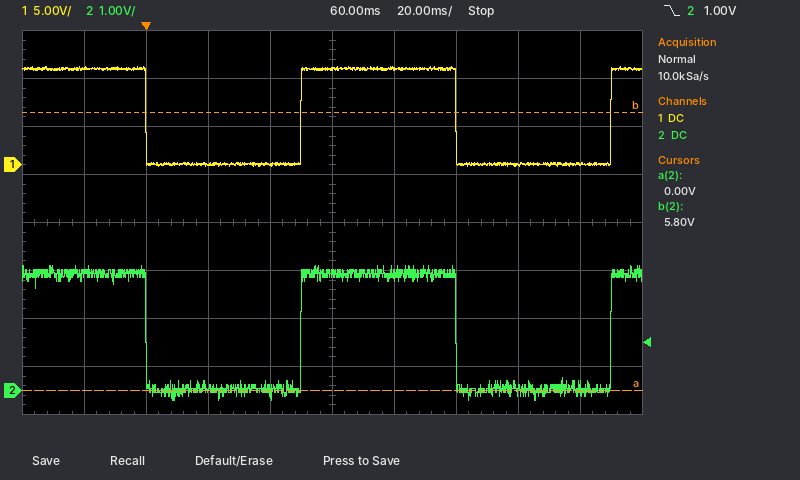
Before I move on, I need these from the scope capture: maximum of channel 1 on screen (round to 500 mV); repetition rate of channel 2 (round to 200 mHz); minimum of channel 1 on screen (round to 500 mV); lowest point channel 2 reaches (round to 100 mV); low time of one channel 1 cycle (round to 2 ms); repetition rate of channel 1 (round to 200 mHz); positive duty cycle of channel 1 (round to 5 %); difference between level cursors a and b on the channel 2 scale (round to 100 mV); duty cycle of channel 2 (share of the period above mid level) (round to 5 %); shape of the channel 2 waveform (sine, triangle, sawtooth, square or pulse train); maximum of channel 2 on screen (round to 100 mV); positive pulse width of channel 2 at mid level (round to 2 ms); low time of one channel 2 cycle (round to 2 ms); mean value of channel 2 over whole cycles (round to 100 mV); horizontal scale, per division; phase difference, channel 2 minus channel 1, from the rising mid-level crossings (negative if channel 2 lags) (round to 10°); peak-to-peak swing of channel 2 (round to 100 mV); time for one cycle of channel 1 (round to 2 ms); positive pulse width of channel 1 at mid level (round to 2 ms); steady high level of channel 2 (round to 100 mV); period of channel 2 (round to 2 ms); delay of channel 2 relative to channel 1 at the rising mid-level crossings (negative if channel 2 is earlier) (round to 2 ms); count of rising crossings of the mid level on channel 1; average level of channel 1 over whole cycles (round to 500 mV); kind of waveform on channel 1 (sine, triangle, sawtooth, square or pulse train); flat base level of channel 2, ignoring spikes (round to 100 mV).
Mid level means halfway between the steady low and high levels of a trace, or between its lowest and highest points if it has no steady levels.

10.0 V
10.0 Hz
0.0 V
-200 mV
50 ms
10.0 Hz
50 %
5.8 V
50 %
square
2.6 V
50 ms
50 ms
1.2 V
20 ms
0°
2.8 V
100 ms
50 ms
2.4 V
100 ms
0 ms
2
5.0 V
square
0.0 V
